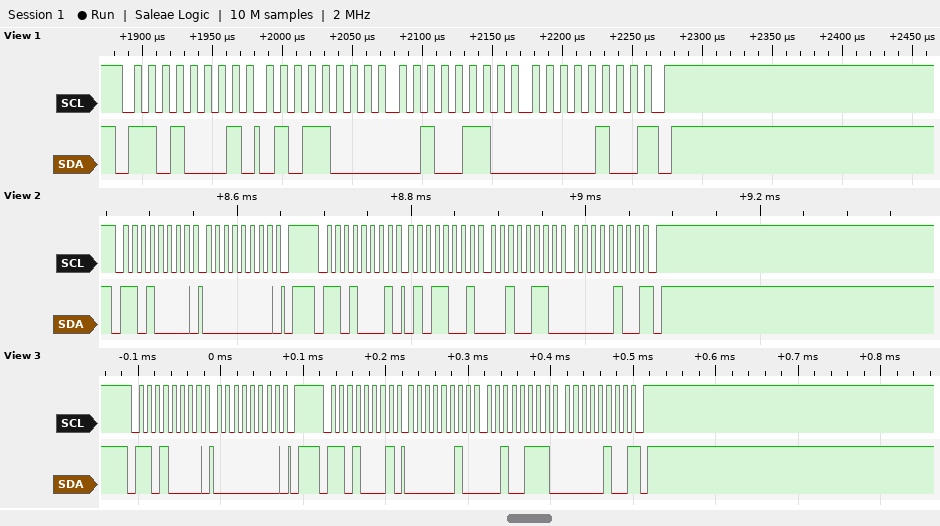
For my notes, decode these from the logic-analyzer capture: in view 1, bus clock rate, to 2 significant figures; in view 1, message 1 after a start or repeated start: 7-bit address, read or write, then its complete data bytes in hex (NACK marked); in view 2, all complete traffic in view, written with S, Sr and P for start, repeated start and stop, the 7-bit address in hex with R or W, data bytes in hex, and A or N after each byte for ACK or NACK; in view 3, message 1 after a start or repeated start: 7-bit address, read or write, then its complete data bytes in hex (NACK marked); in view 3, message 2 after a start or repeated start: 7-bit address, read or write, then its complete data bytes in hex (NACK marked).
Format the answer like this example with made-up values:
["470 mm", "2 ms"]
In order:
["100 kHz", "0x68 read: 58 26 04 NACK", "S 68W A 00 A P S 68R A 59 A 26 A 04 N P", "0x68 write: 00", "0x68 read: 02 27 04 NACK"]
